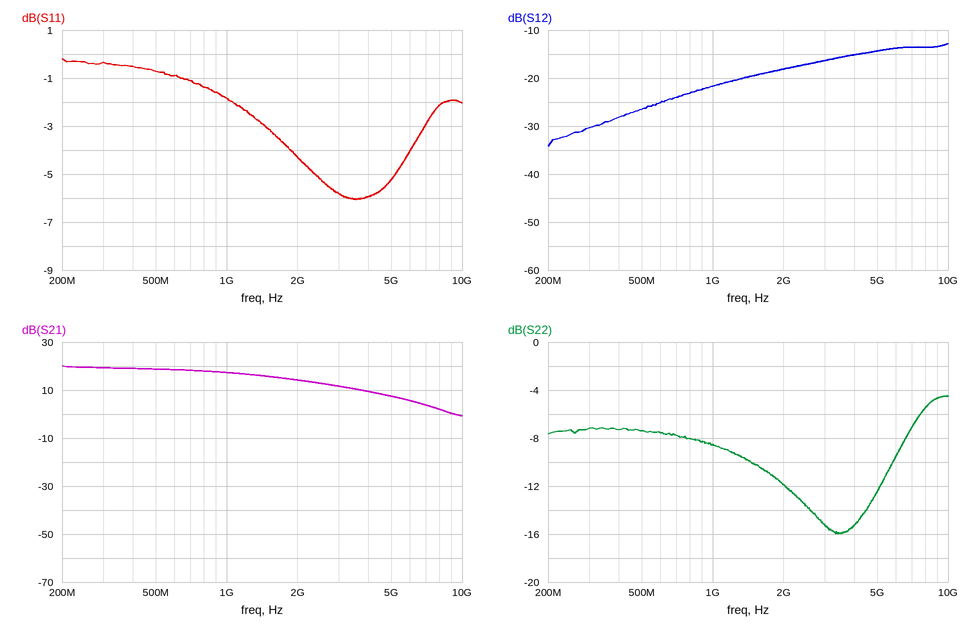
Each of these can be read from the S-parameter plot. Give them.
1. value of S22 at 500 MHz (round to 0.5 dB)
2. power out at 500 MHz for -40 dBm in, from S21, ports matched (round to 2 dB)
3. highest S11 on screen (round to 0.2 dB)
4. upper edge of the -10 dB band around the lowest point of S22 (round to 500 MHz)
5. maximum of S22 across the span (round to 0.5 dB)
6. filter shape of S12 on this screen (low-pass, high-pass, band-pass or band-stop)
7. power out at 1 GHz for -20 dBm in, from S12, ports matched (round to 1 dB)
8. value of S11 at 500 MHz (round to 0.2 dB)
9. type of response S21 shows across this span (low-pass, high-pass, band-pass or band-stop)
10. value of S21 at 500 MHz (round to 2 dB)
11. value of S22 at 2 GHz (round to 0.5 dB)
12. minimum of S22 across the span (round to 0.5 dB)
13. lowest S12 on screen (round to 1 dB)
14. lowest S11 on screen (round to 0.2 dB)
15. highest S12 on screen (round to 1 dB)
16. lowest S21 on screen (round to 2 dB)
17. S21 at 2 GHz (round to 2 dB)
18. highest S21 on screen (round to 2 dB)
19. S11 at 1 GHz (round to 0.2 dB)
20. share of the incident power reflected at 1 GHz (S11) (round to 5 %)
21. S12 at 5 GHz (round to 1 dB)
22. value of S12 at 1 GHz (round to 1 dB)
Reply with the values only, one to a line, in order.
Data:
-7.5 dB
-22 dBm
-0.2 dB
6.0 GHz
-4.5 dB
high-pass
-42 dBm
-0.8 dB
low-pass
18 dB
-12.0 dB
-16.0 dB
-34 dB
-6.0 dB
-13 dB
0 dB
14 dB
20 dB
-1.8 dB
65 %
-14 dB
-22 dB
